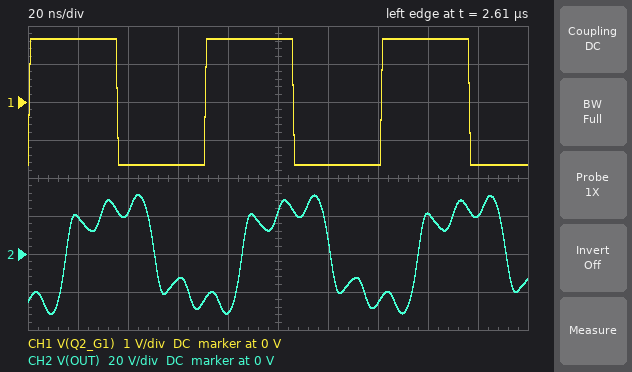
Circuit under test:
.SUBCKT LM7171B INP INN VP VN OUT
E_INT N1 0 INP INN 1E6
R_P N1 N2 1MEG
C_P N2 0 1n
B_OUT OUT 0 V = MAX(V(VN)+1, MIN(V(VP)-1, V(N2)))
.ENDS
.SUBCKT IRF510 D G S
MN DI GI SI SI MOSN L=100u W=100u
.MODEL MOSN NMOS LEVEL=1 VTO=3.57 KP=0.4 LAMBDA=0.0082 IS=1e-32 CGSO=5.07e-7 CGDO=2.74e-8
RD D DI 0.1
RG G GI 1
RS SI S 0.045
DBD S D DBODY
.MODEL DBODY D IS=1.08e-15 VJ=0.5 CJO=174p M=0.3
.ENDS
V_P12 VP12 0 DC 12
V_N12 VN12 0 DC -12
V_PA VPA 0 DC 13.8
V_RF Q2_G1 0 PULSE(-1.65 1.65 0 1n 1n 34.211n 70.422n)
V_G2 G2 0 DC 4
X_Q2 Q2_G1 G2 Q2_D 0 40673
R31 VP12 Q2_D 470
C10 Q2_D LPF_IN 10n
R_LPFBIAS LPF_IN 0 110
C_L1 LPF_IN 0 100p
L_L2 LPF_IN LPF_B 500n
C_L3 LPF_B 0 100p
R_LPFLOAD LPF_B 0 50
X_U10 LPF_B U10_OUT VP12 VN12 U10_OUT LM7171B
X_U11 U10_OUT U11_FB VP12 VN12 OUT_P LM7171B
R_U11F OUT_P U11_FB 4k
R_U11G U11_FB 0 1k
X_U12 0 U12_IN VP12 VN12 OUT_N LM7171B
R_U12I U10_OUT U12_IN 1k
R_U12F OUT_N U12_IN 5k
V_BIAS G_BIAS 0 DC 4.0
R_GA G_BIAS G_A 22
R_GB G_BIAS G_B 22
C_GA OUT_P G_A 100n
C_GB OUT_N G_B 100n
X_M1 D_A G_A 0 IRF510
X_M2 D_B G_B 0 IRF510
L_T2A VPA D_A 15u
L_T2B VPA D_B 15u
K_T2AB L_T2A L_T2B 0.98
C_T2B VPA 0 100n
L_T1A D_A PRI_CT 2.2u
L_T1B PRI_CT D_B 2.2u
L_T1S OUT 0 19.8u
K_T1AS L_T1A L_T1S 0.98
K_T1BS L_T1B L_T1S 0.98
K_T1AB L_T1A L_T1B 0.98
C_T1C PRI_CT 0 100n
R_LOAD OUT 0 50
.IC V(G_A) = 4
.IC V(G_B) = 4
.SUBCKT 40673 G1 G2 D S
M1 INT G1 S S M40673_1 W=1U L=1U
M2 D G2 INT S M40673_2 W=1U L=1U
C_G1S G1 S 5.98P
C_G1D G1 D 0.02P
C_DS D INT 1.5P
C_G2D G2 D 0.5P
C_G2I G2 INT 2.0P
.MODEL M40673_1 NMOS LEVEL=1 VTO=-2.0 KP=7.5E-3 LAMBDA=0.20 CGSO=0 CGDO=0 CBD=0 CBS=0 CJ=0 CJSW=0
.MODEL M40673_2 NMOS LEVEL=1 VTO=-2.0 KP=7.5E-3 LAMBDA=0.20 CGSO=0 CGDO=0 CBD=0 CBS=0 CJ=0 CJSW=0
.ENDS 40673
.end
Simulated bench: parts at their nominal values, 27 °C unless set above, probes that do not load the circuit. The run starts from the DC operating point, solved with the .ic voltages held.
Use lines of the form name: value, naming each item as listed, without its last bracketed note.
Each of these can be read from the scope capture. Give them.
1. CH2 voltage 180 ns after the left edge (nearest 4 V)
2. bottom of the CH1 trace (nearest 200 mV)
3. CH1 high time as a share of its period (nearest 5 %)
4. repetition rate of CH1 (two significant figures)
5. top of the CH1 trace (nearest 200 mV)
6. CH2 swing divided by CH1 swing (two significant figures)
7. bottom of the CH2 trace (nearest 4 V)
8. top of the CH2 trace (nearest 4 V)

CH2 voltage 180 ns after the left edge: 20 V
bottom of the CH1 trace: -1.6 V
CH1 high time as a share of its period: 50 %
repetition rate of CH1: 14 MHz
top of the CH1 trace: 1.6 V
CH2 swing divided by CH1 swing: 19
bottom of the CH2 trace: -32 V
top of the CH2 trace: 32 V
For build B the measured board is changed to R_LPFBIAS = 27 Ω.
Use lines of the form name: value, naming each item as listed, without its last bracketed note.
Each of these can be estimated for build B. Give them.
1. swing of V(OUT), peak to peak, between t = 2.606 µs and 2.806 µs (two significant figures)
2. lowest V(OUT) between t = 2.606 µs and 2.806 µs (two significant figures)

swing of V(OUT), peak to peak, between t = 2.606 µs and 2.806 µs: 36 V
lowest V(OUT) between t = 2.606 µs and 2.806 µs: -19 V
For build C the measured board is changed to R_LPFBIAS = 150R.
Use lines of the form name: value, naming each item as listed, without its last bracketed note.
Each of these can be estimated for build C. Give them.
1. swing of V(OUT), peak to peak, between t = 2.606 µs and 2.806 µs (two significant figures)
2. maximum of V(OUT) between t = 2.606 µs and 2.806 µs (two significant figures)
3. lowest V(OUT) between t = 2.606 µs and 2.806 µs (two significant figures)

swing of V(OUT), peak to peak, between t = 2.606 µs and 2.806 µs: 65 V
maximum of V(OUT) between t = 2.606 µs and 2.806 µs: 32 V
lowest V(OUT) between t = 2.606 µs and 2.806 µs: -33 V
